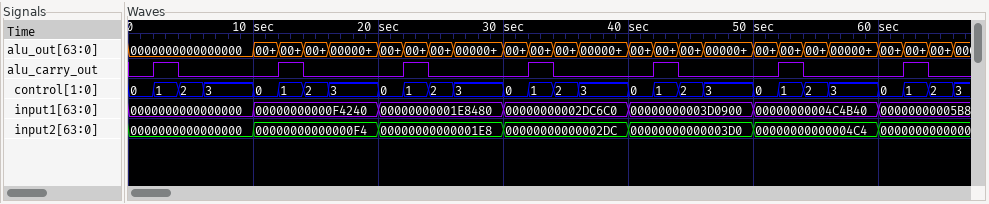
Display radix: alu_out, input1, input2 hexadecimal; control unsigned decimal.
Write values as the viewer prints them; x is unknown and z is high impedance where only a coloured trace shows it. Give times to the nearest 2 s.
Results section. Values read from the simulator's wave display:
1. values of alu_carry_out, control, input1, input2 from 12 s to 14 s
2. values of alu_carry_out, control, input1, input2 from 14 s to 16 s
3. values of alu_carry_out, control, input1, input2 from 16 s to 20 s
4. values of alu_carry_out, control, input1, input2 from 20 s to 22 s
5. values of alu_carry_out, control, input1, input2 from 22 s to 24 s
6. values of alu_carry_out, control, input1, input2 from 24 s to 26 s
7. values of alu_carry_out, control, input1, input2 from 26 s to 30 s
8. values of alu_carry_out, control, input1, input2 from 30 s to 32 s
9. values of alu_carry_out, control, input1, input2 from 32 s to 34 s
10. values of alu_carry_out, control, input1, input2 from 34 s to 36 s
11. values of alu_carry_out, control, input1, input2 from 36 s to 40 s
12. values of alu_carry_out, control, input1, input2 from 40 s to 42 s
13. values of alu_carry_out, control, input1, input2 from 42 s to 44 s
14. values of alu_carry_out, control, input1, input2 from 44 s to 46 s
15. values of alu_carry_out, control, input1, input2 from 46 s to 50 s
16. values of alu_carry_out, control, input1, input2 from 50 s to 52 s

alu_carry_out=1, control=1, input1=00000000000F4240, input2=00000000000000F4
alu_carry_out=0, control=2, input1=00000000000F4240, input2=00000000000000F4
alu_carry_out=0, control=3, input1=00000000000F4240, input2=00000000000000F4
alu_carry_out=0, control=0, input1=00000000001E8480, input2=00000000000001E8
alu_carry_out=1, control=1, input1=00000000001E8480, input2=00000000000001E8
alu_carry_out=0, control=2, input1=00000000001E8480, input2=00000000000001E8
alu_carry_out=0, control=3, input1=00000000001E8480, input2=00000000000001E8
alu_carry_out=0, control=0, input1=00000000002DC6C0, input2=00000000000002DC
alu_carry_out=1, control=1, input1=00000000002DC6C0, input2=00000000000002DC
alu_carry_out=0, control=2, input1=00000000002DC6C0, input2=00000000000002DC
alu_carry_out=0, control=3, input1=00000000002DC6C0, input2=00000000000002DC
alu_carry_out=0, control=0, input1=00000000003D0900, input2=00000000000003D0
alu_carry_out=1, control=1, input1=00000000003D0900, input2=00000000000003D0
alu_carry_out=0, control=2, input1=00000000003D0900, input2=00000000000003D0
alu_carry_out=0, control=3, input1=00000000003D0900, input2=00000000000003D0
alu_carry_out=0, control=0, input1=00000000004C4B40, input2=00000000000004C4
